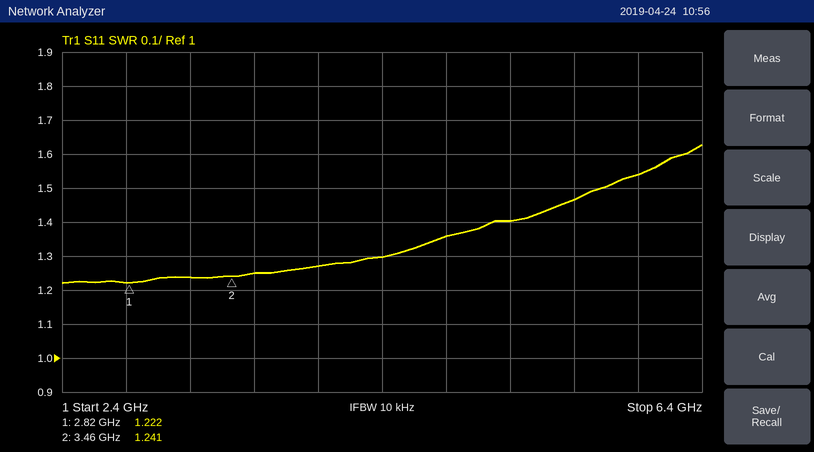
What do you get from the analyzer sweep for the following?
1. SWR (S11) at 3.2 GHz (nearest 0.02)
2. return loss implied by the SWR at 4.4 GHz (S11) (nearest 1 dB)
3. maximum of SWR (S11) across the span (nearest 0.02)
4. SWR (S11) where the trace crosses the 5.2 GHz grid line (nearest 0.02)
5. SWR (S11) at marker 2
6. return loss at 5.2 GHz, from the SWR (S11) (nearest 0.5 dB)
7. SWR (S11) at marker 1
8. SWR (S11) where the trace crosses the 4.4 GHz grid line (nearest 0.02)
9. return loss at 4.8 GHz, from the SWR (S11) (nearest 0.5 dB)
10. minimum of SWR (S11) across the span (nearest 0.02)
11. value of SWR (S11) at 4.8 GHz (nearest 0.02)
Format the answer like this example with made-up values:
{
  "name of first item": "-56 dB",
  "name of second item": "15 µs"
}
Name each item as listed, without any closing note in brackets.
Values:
{
  "SWR (S11) at 3.2 GHz": "1.24",
  "return loss implied by the SWR at 4.4 GHz (S11)": "18 dB",
  "maximum of SWR (S11) across the span": "1.62",
  "SWR (S11) where the trace crosses the 5.2 GHz grid line": "1.40",
  "SWR (S11) at marker 2": "1.241",
  "return loss at 5.2 GHz, from the SWR (S11)": "15.5 dB",
  "SWR (S11) at marker 1": "1.222",
  "SWR (S11) where the trace crosses the 4.4 GHz grid line": "1.30",
  "return loss at 4.8 GHz, from the SWR (S11)": "16.5 dB",
  "minimum of SWR (S11) across the span": "1.22",
  "value of SWR (S11) at 4.8 GHz": "1.36"
}
